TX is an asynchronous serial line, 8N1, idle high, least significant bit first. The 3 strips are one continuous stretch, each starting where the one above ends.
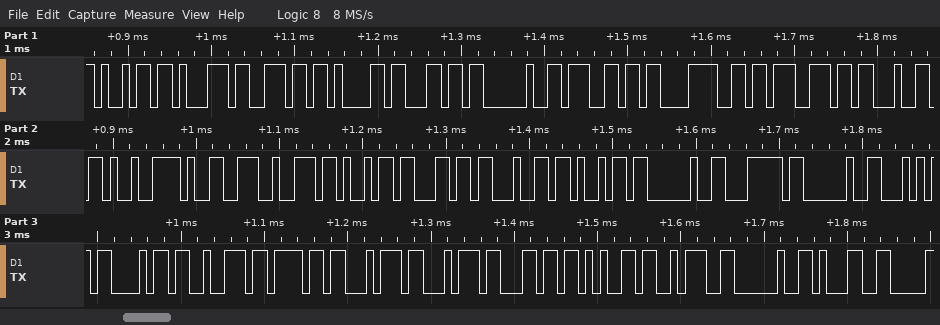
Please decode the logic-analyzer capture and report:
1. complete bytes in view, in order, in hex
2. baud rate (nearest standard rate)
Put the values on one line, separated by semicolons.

69 71 6E 61 6C 20 67 C3 B6 6E 64 C9 99 72 69 6C 64 69 20 7C 20 54 68 72 6F 74 74 6C 65 3A 20 31; 115200 baud
